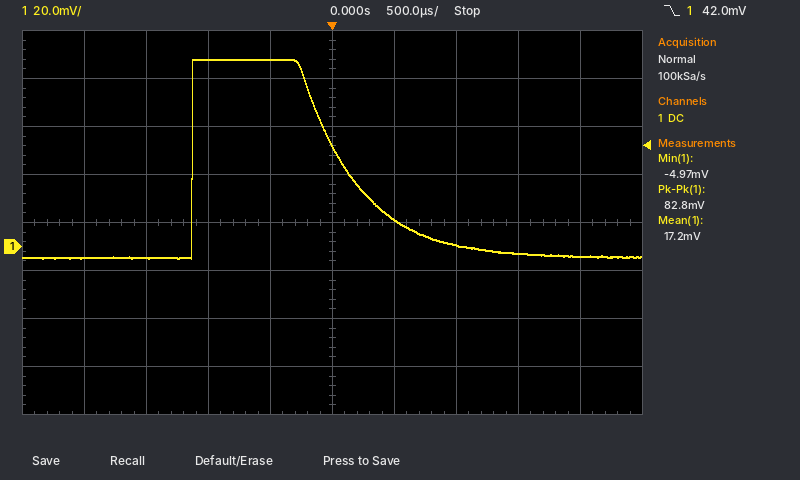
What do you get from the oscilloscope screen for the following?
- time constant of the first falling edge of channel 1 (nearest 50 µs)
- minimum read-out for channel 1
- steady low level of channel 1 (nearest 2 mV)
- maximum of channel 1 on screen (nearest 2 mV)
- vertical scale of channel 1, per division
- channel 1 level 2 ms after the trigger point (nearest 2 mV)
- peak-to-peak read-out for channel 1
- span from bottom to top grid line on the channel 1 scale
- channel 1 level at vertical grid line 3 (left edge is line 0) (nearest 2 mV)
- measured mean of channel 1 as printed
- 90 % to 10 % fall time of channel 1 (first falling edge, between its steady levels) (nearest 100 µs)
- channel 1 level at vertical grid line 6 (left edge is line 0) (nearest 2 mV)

450 µs
-4.97 mV
-4 mV
78 mV
20 mV
-4 mV
82.8 mV
160 mV
78 mV
17.2 mV
1.0 ms
12 mV
